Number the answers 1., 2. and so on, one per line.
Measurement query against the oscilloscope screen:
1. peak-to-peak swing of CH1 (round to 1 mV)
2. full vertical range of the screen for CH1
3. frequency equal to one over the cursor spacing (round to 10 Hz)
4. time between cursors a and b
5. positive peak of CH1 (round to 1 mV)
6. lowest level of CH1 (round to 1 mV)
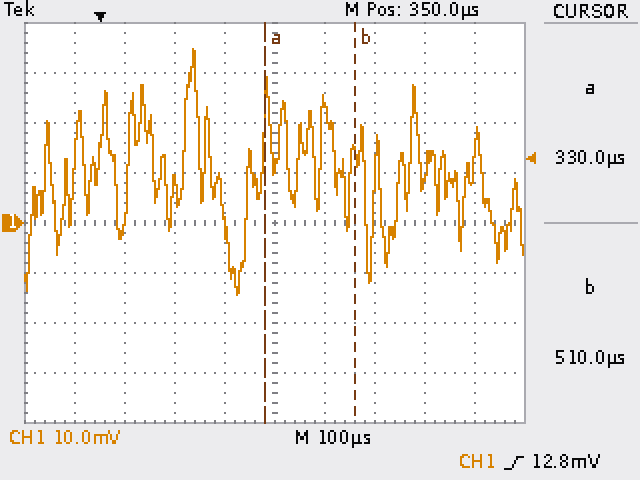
1. 49 mV
2. 80 mV
3. 5.56 kHz
4. 180 µs
5. 35 mV
6. -14 mV
